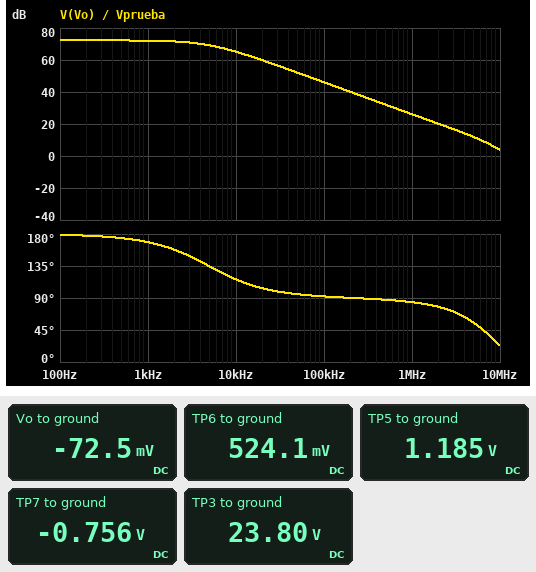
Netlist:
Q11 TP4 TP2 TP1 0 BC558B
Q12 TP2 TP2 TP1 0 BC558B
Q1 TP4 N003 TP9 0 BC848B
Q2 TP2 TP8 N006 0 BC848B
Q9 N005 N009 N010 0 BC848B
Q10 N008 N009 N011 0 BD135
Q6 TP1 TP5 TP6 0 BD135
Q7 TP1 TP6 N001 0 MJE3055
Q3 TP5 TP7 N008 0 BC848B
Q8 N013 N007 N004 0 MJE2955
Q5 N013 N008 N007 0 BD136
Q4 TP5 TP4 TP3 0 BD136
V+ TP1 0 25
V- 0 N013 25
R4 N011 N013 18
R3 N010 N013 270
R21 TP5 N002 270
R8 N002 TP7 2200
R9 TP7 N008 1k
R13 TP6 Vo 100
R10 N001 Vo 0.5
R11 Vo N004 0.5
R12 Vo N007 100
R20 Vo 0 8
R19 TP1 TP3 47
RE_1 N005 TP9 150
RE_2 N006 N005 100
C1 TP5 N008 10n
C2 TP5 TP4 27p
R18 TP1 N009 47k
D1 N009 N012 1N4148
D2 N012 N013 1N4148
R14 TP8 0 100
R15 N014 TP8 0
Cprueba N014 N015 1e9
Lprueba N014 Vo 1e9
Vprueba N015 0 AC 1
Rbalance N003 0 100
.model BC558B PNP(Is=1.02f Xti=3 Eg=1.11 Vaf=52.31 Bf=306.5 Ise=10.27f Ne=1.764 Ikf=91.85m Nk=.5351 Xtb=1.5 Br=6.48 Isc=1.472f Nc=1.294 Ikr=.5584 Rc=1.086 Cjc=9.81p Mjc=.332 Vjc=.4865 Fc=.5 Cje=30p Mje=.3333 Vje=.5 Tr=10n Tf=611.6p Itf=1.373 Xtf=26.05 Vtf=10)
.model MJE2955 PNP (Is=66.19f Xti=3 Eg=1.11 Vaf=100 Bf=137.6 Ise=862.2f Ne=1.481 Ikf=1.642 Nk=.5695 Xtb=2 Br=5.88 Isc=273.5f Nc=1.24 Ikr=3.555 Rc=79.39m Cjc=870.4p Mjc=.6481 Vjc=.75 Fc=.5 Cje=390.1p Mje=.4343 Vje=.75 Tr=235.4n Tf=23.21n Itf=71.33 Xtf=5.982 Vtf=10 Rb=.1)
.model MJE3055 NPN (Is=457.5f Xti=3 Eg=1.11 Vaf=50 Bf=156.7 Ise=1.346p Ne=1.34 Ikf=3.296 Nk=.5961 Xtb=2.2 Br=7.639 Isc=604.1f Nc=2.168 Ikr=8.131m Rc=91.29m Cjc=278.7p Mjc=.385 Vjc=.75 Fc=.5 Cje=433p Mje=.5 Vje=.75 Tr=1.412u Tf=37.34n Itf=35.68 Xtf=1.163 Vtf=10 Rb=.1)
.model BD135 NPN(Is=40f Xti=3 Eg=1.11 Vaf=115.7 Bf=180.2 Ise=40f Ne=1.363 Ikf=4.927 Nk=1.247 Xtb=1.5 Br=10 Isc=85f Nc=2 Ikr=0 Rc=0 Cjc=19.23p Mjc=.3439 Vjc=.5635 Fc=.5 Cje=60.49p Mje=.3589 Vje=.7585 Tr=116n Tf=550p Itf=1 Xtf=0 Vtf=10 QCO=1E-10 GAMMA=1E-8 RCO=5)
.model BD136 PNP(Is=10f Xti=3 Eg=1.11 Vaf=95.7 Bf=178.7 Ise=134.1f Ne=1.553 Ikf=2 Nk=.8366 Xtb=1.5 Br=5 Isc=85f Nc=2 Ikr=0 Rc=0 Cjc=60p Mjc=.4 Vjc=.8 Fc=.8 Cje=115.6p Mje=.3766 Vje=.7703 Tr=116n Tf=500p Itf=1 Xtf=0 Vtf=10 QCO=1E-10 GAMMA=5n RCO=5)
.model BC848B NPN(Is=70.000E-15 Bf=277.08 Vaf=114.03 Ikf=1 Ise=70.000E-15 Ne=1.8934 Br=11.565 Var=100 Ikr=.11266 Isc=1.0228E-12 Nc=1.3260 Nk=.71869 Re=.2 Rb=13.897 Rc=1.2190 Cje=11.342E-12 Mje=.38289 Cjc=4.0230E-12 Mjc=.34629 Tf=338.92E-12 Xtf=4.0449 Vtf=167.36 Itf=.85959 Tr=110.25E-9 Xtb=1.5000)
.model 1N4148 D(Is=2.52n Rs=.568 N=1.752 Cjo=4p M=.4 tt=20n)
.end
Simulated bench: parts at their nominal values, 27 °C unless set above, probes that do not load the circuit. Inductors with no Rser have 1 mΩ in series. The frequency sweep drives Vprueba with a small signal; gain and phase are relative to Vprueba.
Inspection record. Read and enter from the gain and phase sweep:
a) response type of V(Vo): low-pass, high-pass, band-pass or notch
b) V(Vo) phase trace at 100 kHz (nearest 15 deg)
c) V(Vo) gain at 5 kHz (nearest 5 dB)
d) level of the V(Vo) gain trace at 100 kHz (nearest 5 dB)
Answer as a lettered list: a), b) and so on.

a) low-pass
b) 90 deg
c) 70 dB
d) 45 dB
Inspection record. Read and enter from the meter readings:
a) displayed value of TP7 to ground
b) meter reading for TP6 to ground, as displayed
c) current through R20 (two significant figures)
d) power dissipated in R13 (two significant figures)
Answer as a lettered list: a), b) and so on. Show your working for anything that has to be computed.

a) -0.756 V
b) 524.1 mV
c) (0 V - (-72.5 mV)) / 8 Ω = 9.1 mA
d) (524.1 mV - (-72.5 mV))^2 / 100 Ω = 3.6 mW
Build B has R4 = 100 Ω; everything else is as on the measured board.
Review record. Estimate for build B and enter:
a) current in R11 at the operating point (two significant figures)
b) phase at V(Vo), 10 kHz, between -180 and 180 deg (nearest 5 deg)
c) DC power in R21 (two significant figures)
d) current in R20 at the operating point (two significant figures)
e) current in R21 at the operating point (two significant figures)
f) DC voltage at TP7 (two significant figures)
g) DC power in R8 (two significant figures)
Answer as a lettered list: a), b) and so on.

a) 4.0 mA
b) 100 deg
c) 120 µW
d) 6.9 mA
e) 660 µA
f) -750 mV
g) 960 µW
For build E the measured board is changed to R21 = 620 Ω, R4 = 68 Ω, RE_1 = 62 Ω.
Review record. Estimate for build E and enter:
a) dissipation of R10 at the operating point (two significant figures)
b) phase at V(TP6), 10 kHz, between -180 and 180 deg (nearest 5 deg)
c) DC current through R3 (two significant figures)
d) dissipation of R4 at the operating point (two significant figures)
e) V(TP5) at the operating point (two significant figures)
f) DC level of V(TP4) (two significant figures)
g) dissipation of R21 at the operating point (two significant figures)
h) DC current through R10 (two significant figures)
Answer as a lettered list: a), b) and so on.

a) 22 µW
b) 100 deg
c) 2.0 mA
d) 3.7 mW
e) 1.3 V
f) 24 V
g) 290 µW
h) 6.6 mA
